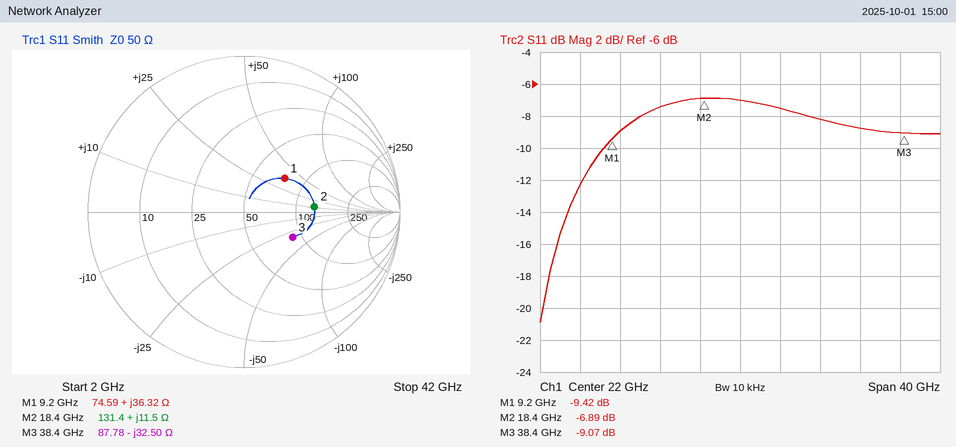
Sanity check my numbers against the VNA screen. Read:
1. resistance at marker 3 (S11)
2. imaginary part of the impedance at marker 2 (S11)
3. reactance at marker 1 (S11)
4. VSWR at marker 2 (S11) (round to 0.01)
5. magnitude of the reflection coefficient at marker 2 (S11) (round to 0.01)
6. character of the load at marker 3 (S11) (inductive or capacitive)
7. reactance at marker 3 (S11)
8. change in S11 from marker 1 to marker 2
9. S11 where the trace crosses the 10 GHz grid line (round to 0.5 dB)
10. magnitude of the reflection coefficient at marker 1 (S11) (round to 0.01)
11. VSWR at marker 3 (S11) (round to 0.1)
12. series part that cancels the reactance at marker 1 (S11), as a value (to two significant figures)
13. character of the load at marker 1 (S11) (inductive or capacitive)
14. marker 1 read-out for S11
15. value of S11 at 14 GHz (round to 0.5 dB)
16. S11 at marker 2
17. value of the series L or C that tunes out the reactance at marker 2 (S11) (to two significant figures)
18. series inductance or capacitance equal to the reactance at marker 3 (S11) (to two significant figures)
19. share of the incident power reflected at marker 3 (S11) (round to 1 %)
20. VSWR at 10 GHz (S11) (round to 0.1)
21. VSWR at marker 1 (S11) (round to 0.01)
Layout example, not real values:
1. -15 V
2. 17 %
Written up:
1. 87.78 Ω
2. +11.5 Ω
3. +36.32 Ω
4. 2.65
5. 0.45
6. capacitive
7. -32.50 Ω
8. 2.53 dB
9. -9.0 dB
10. 0.34
11. 2.1
12. 480 fF
13. inductive
14. -9.42 dB
15. -7.5 dB
16. -6.89 dB
17. 750 fF
18. 130 fF
19. 12 %
20. 2.1
21. 2.02
